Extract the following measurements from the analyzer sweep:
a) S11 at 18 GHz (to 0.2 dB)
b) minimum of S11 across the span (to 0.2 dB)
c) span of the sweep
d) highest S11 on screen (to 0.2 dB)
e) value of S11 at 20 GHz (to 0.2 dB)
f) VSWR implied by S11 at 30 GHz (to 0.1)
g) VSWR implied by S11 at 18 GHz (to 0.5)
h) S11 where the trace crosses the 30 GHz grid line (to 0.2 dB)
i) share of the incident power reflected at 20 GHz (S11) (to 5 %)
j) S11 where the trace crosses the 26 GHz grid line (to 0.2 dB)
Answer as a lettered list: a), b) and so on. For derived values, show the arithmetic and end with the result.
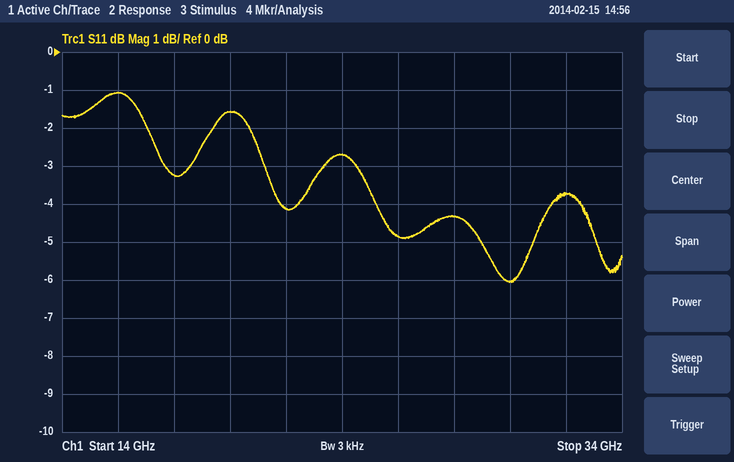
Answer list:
a) -3.2 dB
b) -6.0 dB
c) 20 GHz
d) -1.0 dB
e) -1.6 dB
f) |Γ| = 10^(-6/20) = 0.5012; VSWR = (1 + 0.5012)/(1 − 0.5012) ≈ 3.0
g) |Γ| = 10^(-3.2/20) = 0.6918; VSWR = (1 + 0.6918)/(1 − 0.6918) ≈ 5.5
h) -6.0 dB
i) 10^(-1.6/10) ≈ 69.2 %, so 70 % to the nearest 5 %
j) -4.8 dB
